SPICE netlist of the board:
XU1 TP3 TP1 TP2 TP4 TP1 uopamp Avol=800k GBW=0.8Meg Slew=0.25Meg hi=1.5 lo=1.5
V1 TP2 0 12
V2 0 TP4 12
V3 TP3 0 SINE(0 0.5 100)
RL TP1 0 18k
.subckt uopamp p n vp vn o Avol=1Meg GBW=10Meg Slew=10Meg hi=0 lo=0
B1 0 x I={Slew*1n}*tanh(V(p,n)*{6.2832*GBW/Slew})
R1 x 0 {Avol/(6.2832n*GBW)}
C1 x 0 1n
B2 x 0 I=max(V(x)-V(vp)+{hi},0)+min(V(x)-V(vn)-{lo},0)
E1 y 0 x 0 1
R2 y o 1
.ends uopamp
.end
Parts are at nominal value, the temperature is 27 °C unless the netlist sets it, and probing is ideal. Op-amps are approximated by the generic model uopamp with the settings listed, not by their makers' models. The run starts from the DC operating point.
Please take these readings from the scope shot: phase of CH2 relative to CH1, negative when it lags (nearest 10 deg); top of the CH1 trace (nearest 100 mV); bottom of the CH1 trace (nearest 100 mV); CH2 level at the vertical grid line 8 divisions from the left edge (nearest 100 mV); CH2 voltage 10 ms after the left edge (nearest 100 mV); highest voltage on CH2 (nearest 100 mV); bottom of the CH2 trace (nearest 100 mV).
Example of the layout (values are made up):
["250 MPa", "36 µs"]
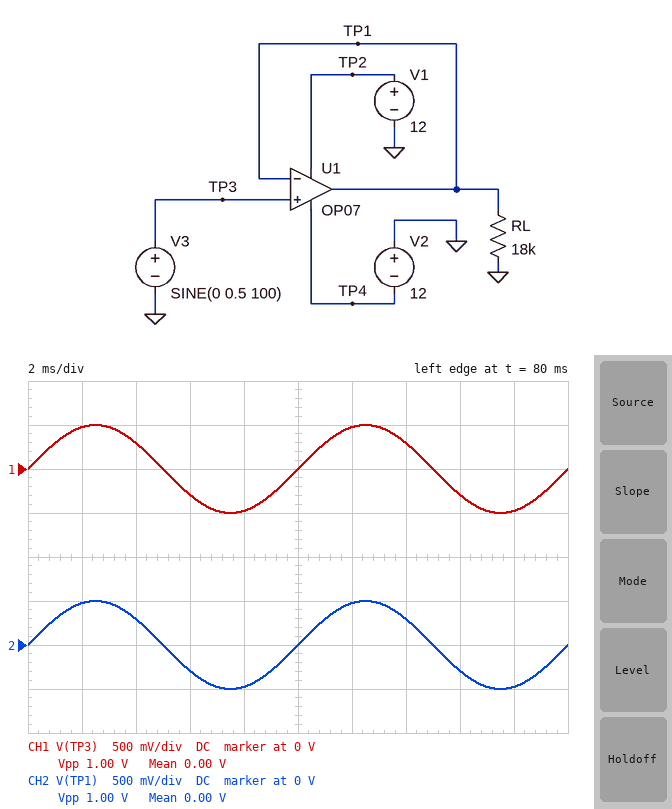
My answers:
["0 deg", "500 mV", "-500 mV", "-300 mV", "0 V", "500 mV", "-500 mV"]
